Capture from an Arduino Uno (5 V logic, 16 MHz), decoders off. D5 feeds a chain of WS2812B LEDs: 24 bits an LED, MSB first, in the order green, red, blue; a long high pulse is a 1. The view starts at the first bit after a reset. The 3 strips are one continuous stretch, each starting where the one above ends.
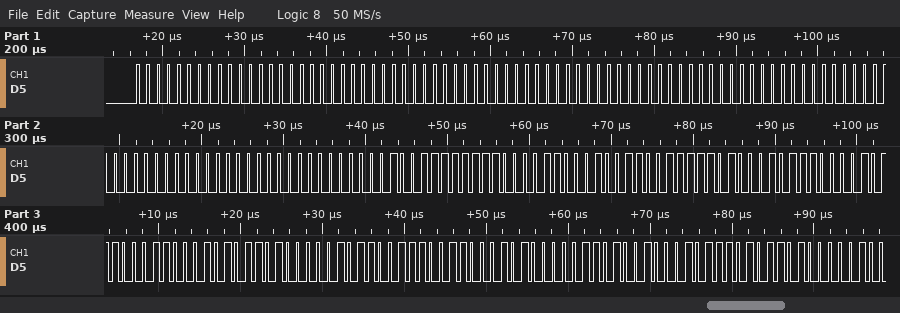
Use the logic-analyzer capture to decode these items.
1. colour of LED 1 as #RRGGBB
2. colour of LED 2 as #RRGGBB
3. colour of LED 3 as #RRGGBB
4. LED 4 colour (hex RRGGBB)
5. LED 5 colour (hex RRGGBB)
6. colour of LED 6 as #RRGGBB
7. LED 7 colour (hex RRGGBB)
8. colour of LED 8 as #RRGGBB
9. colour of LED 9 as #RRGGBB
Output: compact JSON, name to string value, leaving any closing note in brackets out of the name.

{"colour of LED 1 as #RRGGBB": "#000000", "colour of LED 2 as #RRGGBB": "#000000", "colour of LED 3 as #RRGGBB": "#000000", "LED 4 colour": "#000000", "LED 5 colour": "#FF040C", "colour of LED 6 as #RRGGBB": "#FA4C2E", "LED 7 colour": "#31165A", "colour of LED 8 as #RRGGBB": "#390B8A", "colour of LED 9 as #RRGGBB": "#220DEB"}
